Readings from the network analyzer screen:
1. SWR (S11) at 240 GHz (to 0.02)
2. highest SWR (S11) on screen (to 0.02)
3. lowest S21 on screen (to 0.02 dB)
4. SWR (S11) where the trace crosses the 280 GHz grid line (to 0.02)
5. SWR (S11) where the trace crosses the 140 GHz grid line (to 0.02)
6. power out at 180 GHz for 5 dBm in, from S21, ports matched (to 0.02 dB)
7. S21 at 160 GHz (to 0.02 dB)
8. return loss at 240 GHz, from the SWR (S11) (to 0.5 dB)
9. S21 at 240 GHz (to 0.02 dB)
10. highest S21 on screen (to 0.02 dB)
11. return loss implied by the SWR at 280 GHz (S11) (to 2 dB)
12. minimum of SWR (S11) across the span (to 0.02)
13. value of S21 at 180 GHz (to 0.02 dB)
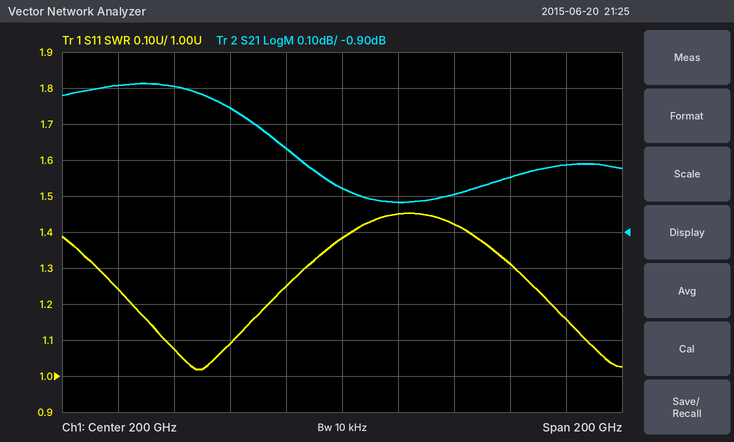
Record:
1.42
1.46
-0.82 dB
1.16
1.08
4.34 dBm
-0.56 dB
15.0 dB
-0.80 dB
-0.48 dB
22 dB
1.02
-0.66 dB
